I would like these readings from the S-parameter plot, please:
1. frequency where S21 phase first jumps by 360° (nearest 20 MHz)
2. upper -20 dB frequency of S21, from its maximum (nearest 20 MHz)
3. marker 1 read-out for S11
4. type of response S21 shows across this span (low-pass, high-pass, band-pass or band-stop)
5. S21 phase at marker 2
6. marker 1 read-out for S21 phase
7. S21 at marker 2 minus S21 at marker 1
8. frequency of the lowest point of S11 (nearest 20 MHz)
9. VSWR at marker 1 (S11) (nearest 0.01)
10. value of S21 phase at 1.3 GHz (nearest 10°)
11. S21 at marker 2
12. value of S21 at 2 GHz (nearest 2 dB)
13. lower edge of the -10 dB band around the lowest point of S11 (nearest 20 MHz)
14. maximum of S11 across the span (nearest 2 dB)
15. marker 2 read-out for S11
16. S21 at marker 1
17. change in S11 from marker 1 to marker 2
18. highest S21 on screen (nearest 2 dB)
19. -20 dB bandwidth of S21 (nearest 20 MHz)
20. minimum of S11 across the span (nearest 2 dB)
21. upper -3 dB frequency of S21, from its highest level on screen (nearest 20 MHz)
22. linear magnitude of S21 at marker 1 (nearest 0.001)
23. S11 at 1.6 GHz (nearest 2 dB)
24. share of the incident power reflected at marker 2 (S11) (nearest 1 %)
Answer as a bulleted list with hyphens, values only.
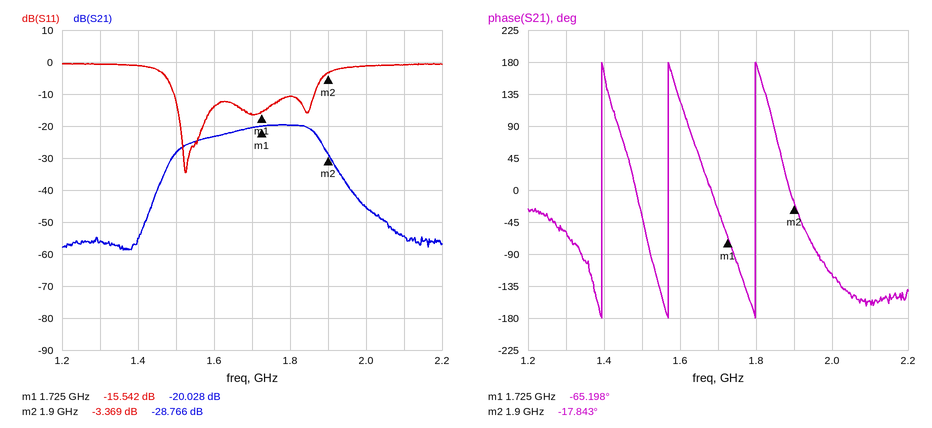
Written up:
- 1.40 GHz
- 1.96 GHz
- -15.542 dB
- band-pass
- -17.843°
- -65.198°
- -8.738 dB
- 1.52 GHz
- 1.40
- -60°
- -28.766 dB
- -46 dB
- 1.50 GHz
- 0 dB
- -3.369 dB
- -20.028 dB
- 12.173 dB
- -20 dB
- 500 MHz
- -34 dB
- 1.86 GHz
- 0.100
- -14 dB
- 46 %
